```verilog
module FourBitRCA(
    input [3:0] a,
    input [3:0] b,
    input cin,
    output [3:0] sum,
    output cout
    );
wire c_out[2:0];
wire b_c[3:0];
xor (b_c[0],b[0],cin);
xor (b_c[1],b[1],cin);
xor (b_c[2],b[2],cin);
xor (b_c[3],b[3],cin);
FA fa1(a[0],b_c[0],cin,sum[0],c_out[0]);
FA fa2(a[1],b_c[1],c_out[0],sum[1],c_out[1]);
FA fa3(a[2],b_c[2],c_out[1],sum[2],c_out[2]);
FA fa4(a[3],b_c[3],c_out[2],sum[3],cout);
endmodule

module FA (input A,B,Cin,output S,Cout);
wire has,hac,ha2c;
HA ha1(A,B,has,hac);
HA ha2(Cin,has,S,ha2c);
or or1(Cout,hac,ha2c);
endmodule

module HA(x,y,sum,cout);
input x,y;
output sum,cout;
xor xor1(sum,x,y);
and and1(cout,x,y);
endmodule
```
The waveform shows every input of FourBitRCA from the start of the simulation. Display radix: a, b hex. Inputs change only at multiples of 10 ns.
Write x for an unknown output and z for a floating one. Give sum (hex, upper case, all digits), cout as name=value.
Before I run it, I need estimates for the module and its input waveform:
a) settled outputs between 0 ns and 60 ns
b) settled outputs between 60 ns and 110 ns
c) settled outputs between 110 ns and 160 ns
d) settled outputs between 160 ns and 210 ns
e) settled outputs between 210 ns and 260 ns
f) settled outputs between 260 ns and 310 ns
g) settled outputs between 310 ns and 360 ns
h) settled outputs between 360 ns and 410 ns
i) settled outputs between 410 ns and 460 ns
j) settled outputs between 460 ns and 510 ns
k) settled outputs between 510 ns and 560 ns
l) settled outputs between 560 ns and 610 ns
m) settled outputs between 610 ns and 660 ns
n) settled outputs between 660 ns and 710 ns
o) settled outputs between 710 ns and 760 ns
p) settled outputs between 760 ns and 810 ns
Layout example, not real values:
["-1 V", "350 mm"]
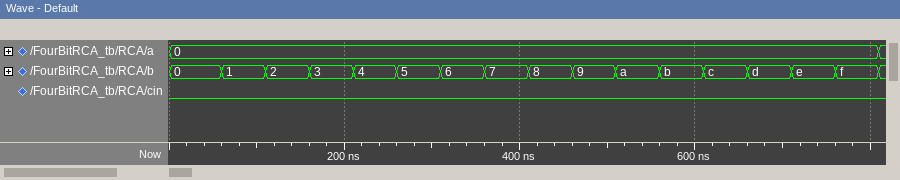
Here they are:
["sum=0, cout=0", "sum=1, cout=0", "sum=2, cout=0", "sum=3, cout=0", "sum=4, cout=0", "sum=5, cout=0", "sum=6, cout=0", "sum=7, cout=0", "sum=8, cout=0", "sum=9, cout=0", "sum=A, cout=0", "sum=B, cout=0", "sum=C, cout=0", "sum=D, cout=0", "sum=E, cout=0", "sum=F, cout=0"]
